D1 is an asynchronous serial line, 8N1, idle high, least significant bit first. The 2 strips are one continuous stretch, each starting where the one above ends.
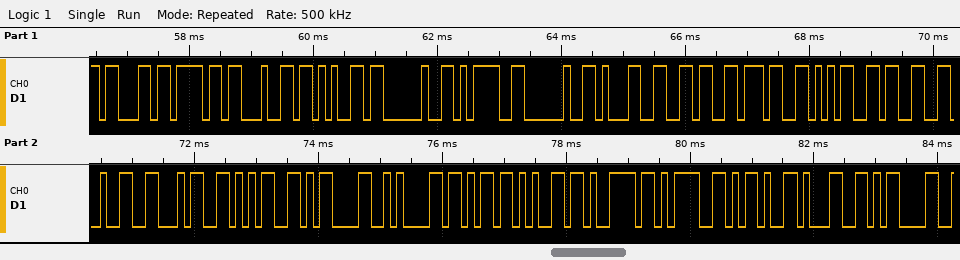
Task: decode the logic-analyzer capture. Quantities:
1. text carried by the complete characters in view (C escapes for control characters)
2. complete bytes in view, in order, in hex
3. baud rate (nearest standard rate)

"code = 16753245\r\nkey=-1\r"
63 6F 64 65 20 3D 20 31 36 37 35 33 32 34 35 0D 0A 6B 65 79 3D 2D 31 0D
9600 baud
